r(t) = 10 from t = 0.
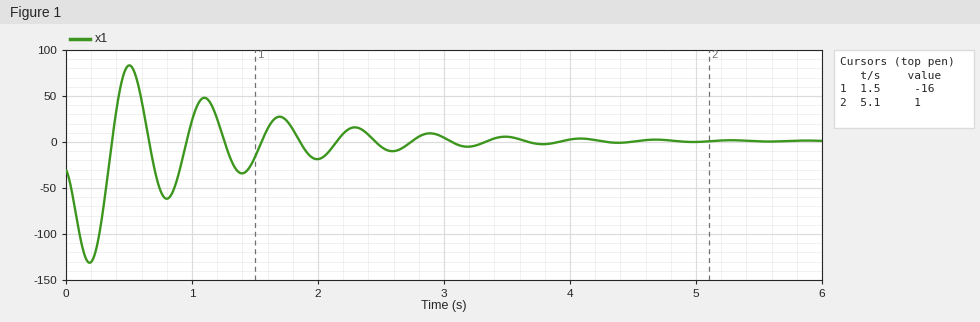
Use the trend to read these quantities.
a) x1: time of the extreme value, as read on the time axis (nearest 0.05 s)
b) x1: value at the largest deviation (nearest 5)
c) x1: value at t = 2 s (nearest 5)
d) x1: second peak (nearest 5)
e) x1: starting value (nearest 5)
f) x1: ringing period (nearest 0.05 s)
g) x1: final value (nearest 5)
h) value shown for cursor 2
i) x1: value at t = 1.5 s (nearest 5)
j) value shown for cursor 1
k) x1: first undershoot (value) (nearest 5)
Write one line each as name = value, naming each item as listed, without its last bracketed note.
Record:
x1: time of the extreme value, as read on the time axis = 0.50 s
x1: value at the largest deviation = 85
x1: value at t = 2 s = -20
x1: second peak = 50
x1: starting value = -30
x1: ringing period = 0.60 s
x1: final value = 0
value shown for cursor 2 = 1
x1: value at t = 1.5 s = -15
value shown for cursor 1 = -16
x1: first undershoot (value) = -60
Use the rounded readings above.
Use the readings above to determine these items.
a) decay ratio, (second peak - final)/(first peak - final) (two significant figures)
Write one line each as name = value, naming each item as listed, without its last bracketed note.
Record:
decay ratio, (second peak - final)/(first peak - final) = 0.59
